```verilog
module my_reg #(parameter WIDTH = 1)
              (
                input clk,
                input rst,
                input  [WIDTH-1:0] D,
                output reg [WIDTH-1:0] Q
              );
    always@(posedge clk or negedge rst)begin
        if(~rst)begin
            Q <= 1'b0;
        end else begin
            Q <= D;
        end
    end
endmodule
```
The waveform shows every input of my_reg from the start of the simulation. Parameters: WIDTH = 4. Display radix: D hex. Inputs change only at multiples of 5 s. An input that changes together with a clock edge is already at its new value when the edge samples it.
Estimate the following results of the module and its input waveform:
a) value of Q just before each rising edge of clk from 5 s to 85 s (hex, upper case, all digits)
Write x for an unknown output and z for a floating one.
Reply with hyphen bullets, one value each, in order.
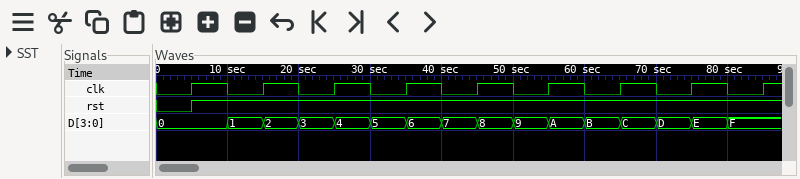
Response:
- 0, 0, 2, 4, 6, 8, A, C, E
